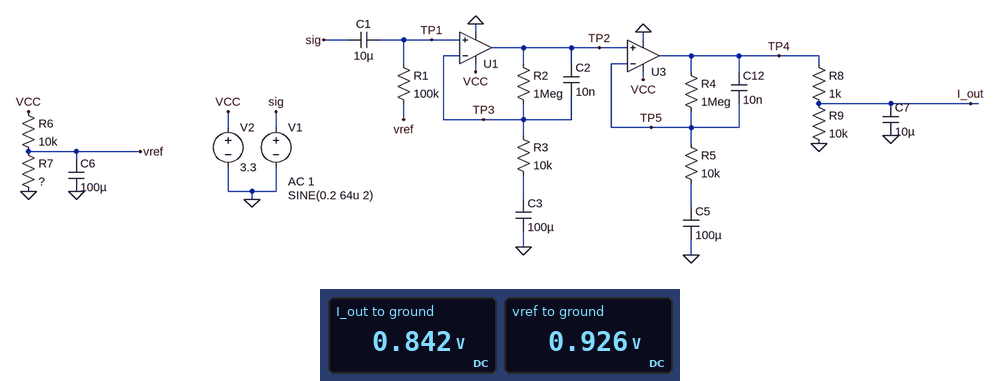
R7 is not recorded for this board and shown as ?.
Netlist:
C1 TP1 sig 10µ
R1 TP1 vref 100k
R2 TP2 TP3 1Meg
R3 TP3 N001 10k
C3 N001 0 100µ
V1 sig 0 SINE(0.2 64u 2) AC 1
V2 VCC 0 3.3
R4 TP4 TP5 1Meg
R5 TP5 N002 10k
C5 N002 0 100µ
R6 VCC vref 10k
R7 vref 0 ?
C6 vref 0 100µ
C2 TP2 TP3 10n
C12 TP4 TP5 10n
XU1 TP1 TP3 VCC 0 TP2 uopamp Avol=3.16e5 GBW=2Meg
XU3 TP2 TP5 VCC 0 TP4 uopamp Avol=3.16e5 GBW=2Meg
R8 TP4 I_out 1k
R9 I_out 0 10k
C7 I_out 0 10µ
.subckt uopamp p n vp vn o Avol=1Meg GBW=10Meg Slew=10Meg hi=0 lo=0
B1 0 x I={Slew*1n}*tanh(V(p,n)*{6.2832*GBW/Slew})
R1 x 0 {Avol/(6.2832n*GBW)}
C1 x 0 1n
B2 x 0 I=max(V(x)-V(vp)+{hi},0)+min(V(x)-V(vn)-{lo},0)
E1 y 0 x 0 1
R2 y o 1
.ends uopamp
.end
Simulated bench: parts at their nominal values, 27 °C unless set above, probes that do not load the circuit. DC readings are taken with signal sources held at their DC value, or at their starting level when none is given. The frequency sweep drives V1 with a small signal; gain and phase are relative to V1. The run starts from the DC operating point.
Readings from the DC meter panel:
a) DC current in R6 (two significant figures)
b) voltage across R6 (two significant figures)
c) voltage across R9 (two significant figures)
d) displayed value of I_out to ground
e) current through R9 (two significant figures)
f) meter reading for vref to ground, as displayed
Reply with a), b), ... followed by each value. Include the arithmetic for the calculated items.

a) (3.3 V - 926 mV) / 10 kΩ = 240 µA
b) 3.3 V - 926 mV = 2.4 V
c) 842 mV = 840 mV
d) 0.842 V
e) (842 mV) / 10 kΩ = 84 µA
f) 0.926 V
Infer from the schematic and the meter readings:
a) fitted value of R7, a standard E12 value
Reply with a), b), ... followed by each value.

a) 3.9 kΩ
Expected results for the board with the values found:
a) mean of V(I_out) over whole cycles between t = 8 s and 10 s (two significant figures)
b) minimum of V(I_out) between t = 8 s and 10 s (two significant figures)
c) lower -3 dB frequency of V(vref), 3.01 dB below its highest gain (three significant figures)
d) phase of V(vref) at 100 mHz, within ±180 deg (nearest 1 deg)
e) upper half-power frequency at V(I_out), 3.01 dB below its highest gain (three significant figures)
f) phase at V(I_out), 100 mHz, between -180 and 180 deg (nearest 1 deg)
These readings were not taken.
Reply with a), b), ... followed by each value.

a) 840 mV
b) 270 mV
c) 106 mHz
d) 47 deg
e) 8.75 Hz
f) 170 deg
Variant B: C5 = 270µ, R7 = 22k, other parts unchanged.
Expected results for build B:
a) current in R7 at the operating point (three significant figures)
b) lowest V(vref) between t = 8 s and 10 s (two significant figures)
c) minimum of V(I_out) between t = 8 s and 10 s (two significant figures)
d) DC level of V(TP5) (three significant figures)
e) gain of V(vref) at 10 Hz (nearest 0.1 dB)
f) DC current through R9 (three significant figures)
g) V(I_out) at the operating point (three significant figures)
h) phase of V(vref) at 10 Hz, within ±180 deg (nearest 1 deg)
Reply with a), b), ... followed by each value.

a) 103 µA
b) 2.3 V
c) 1.5 V
d) 2.27 V
e) -56.0 dB
f) 206 µA
g) 2.06 V
h) -88 deg
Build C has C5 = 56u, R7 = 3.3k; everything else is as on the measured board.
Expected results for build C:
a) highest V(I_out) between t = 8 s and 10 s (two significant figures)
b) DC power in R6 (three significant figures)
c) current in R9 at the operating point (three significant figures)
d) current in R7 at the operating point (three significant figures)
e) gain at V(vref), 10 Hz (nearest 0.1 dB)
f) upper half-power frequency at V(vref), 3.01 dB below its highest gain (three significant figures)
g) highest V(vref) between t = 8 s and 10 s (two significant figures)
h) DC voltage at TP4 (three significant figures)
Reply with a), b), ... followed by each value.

a) 1.3 V
b) 616 µW
c) 74.4 µA
d) 248 µA
e) -56.0 dB
f) 927 mHz
g) 820 mV
h) 819 mV
